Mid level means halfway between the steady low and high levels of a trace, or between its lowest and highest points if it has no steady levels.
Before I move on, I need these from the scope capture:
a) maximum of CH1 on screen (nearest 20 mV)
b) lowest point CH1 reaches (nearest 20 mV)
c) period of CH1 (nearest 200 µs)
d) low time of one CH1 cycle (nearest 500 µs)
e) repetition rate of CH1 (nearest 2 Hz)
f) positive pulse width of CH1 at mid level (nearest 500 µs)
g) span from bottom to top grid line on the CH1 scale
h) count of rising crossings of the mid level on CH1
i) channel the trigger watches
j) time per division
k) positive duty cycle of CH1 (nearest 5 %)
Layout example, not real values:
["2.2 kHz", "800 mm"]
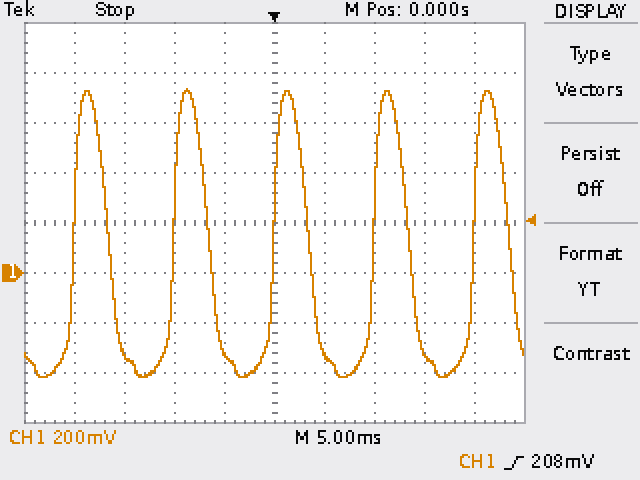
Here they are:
["740 mV", "-420 mV", "10.0 ms", "6.5 ms", "100 Hz", "3.5 ms", "1.6 V", "5", "CH1", "5 ms", "35 %"]
